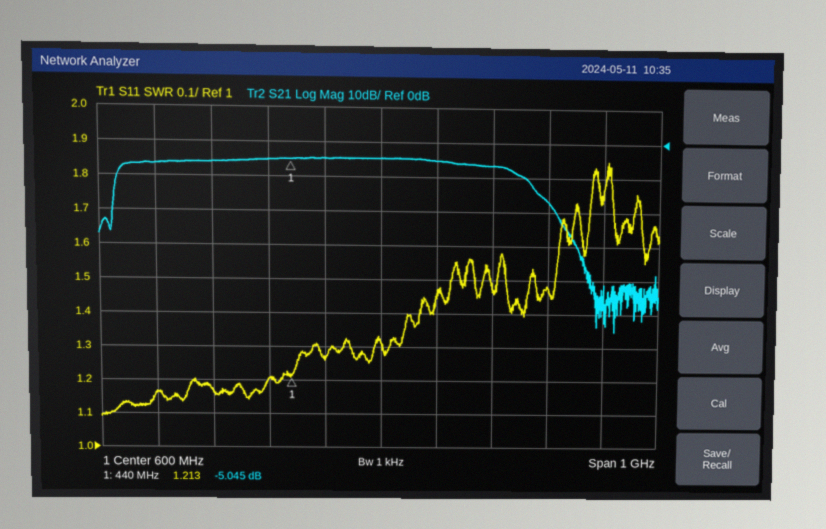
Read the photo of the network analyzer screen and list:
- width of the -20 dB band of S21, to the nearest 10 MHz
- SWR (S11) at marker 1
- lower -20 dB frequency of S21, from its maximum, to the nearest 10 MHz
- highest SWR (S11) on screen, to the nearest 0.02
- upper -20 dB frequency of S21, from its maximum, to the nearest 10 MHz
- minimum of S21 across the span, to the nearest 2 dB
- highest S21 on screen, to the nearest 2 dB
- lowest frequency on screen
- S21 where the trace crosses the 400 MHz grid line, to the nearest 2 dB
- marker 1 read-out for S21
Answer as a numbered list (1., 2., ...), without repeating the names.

1. 810 MHz
2. 1.213
3. 120 MHz
4. 1.84
5. 930 MHz
6. -56 dB
7. -4 dB
8. 100 MHz
9. -6 dB
10. -5.045 dB
